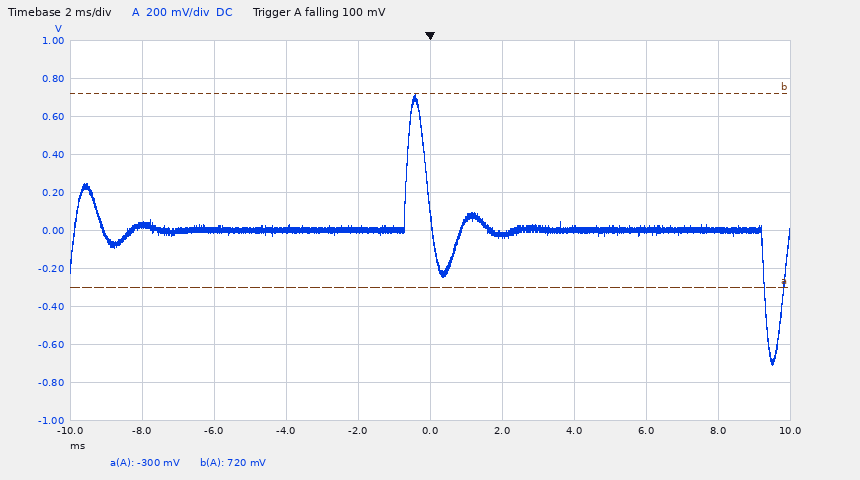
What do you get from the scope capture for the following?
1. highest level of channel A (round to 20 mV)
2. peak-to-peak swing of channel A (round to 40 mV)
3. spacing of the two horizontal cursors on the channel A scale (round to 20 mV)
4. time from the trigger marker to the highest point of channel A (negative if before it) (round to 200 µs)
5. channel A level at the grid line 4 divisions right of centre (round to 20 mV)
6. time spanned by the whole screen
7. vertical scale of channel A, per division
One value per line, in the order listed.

720 mV
1.44 V
1.02 V
-400 µs
0 mV
20 ms
200 mV
